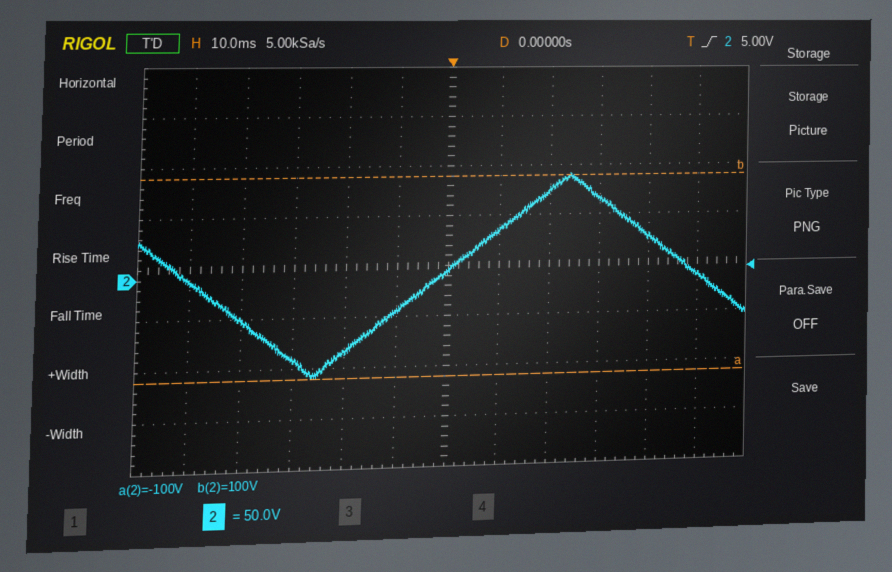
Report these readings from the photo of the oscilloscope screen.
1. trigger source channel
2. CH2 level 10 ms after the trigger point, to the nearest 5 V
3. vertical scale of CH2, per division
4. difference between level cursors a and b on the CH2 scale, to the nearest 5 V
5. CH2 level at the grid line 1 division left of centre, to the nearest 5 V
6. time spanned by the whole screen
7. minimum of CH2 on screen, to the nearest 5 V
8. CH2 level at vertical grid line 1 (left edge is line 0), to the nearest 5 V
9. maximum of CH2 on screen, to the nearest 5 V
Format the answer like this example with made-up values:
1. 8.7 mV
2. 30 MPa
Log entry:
1. CH2
2. 45 V
3. 50 V
4. 200 V
5. -35 V
6. 120 ms
7. -100 V
8. 0 V
9. 100 V
